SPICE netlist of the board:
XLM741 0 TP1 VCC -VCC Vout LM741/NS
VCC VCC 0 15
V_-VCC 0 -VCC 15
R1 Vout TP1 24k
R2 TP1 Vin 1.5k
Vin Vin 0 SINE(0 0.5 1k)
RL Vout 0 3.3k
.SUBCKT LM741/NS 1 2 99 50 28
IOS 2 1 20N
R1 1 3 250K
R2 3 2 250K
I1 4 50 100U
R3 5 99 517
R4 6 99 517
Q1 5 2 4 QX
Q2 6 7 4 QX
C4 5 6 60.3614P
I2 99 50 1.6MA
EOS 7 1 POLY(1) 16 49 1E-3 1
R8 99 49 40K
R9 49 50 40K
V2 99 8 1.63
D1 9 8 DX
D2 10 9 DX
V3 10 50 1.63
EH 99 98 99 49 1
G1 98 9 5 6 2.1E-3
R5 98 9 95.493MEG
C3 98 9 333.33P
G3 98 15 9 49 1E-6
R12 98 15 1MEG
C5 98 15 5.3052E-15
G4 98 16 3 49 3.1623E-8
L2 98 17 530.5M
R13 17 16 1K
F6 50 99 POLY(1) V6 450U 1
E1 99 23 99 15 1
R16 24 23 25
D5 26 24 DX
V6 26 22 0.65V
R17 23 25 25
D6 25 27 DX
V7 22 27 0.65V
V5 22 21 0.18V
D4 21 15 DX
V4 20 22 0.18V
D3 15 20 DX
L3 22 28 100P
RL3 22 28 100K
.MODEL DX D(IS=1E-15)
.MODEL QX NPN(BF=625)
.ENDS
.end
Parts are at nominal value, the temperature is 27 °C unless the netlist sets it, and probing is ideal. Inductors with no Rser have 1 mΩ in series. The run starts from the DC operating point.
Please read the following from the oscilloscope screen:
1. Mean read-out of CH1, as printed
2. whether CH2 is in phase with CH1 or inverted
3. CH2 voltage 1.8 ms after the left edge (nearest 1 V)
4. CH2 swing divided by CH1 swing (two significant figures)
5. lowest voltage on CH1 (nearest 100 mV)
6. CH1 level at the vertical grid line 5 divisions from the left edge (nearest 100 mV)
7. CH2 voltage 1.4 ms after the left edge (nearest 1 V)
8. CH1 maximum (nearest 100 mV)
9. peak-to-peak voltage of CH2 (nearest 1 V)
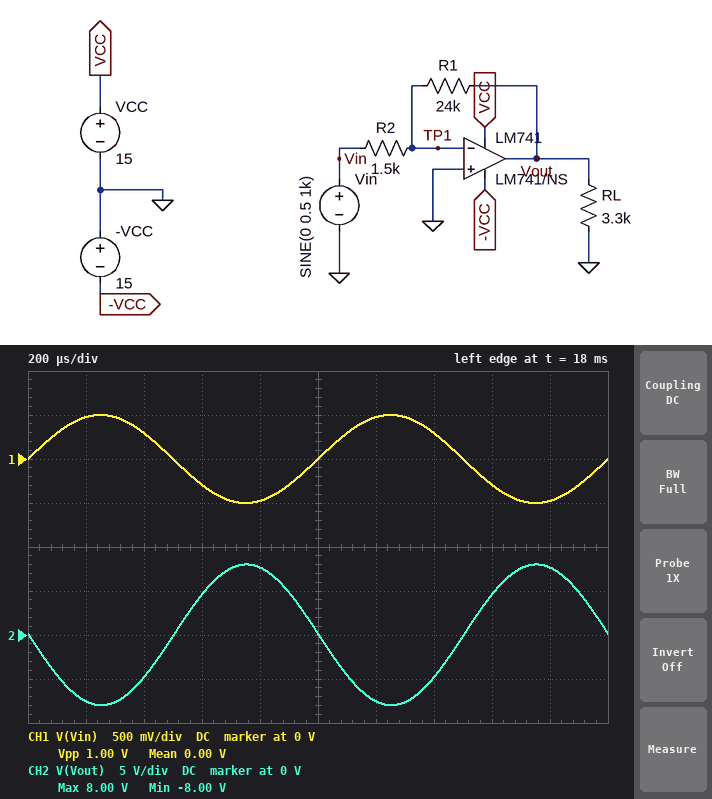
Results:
0.00 V
inverted
8 V
16
-500 mV
0 V
-5 V
500 mV
16 V
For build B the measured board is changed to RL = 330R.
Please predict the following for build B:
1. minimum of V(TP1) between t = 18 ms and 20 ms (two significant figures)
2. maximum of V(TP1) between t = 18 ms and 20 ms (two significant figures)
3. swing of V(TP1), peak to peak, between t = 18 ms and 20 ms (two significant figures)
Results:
-19 mV
22 mV
41 mV
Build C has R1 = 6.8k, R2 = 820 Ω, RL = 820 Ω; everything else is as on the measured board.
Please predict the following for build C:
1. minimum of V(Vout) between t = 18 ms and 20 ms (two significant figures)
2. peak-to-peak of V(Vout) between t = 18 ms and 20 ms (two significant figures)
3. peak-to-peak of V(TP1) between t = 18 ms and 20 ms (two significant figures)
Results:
-4.1 V
8.3 V
10 mV
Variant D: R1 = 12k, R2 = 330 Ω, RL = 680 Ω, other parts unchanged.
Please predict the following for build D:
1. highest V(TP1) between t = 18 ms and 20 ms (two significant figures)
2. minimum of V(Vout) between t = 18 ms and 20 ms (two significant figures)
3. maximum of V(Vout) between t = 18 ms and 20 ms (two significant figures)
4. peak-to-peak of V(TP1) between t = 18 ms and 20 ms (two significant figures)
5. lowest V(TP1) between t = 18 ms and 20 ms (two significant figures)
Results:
130 mV
-13 V
13 V
260 mV
-130 mV
